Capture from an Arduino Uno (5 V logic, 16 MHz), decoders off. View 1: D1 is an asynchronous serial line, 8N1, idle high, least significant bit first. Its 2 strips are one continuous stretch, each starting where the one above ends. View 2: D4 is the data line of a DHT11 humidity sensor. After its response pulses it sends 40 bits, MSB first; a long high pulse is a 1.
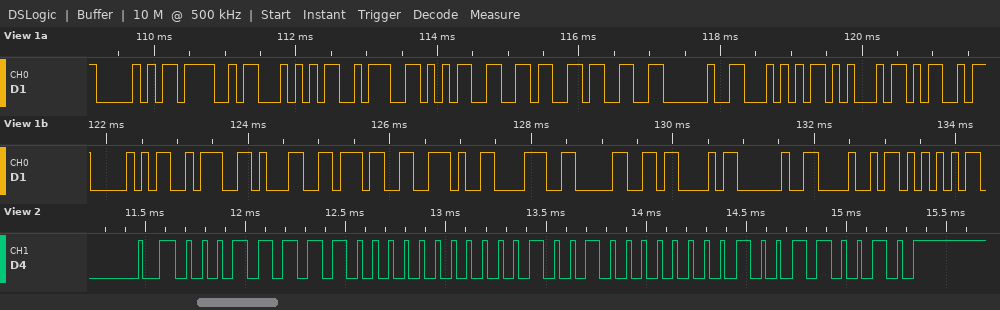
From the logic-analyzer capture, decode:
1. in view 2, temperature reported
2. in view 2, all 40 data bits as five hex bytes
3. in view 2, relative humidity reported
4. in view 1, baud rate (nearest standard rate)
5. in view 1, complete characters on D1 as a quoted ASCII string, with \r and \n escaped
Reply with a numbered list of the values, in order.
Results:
1. 18.1 °C
2. 1F 00 12 01 32
3. 31 %
4. 9600 baud
5. "POT:563 TEMP:17.80C HU"
